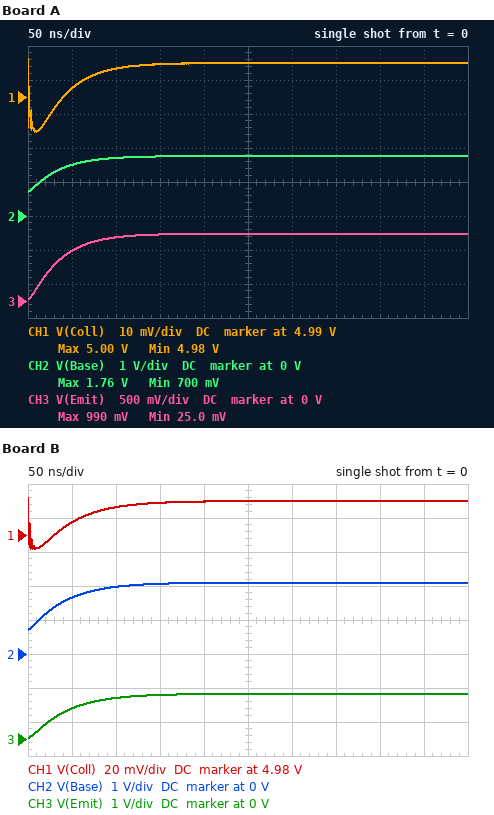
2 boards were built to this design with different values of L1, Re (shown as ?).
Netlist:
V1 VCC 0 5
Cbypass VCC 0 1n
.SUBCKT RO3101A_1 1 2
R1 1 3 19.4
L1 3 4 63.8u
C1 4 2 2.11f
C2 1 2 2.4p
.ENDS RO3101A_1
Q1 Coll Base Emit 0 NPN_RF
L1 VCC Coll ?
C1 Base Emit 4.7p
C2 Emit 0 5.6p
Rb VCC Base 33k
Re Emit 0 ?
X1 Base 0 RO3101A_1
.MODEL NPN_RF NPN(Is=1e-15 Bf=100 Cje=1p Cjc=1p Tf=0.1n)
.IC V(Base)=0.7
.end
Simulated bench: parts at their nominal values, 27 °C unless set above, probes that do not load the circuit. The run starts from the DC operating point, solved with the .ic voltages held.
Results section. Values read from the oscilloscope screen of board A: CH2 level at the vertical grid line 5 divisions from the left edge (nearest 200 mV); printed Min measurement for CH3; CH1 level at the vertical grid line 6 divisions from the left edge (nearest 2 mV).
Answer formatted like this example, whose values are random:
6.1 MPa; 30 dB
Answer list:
1.8 V; 25.0 mV; 5.000 V
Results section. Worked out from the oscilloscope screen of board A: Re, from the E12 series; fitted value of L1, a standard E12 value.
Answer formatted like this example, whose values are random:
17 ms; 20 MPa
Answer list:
100 Ω; 100 nH
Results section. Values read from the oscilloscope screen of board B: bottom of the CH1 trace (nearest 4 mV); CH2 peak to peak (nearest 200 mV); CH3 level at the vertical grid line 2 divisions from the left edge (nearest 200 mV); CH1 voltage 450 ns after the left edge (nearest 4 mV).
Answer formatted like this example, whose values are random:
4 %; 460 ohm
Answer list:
4.972 V; 1.4 V; 1.2 V; 5.000 V
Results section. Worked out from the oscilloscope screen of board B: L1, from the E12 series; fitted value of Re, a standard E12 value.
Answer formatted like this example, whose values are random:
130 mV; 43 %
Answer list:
180 nH; 150 Ω
